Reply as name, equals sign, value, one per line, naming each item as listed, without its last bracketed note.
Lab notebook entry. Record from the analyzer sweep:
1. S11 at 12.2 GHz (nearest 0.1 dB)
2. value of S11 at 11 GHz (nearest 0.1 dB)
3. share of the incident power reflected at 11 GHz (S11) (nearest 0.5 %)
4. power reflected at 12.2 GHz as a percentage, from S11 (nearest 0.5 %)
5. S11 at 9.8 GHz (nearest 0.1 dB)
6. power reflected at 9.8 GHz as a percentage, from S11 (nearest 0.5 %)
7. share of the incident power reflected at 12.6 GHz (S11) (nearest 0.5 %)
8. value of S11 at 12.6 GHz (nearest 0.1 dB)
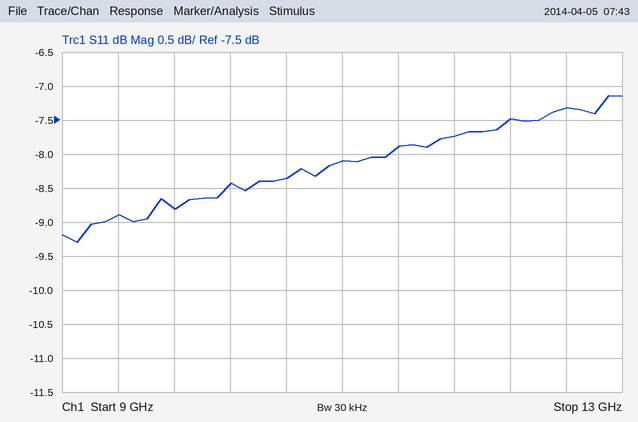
S11 at 12.2 GHz = -7.5 dB
value of S11 at 11 GHz = -8.1 dB
share of the incident power reflected at 11 GHz (S11) = 15.5 %
power reflected at 12.2 GHz as a percentage, from S11 = 18.0 %
S11 at 9.8 GHz = -8.8 dB
power reflected at 9.8 GHz as a percentage, from S11 = 13.0 %
share of the incident power reflected at 12.6 GHz (S11) = 18.5 %
value of S11 at 12.6 GHz = -7.3 dB
